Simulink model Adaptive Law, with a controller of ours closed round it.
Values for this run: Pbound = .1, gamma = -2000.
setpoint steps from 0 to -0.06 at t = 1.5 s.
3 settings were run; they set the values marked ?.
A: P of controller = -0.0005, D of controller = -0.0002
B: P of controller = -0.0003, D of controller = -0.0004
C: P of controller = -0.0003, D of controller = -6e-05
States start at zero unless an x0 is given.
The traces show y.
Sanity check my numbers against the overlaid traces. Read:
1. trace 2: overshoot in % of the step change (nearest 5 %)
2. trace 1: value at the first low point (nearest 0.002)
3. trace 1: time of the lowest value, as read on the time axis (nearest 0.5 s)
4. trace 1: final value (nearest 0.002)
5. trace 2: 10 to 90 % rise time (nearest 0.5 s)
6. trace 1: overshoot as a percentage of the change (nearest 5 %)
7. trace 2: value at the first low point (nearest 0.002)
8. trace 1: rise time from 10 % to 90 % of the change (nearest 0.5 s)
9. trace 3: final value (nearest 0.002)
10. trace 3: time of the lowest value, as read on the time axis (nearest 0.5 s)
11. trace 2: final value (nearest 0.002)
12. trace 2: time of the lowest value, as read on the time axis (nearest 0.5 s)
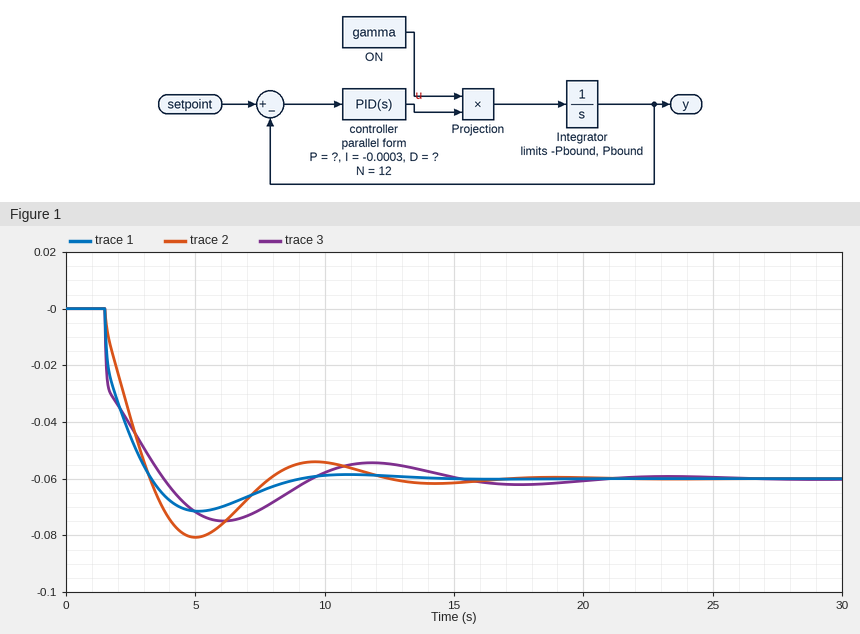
35 %
-0.072
5.0 s
-0.060
1.5 s
20 %
-0.080
1.5 s
-0.060
6.0 s
-0.060
5.0 s
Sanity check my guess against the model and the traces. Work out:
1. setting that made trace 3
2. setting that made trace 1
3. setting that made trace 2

B
A
C
